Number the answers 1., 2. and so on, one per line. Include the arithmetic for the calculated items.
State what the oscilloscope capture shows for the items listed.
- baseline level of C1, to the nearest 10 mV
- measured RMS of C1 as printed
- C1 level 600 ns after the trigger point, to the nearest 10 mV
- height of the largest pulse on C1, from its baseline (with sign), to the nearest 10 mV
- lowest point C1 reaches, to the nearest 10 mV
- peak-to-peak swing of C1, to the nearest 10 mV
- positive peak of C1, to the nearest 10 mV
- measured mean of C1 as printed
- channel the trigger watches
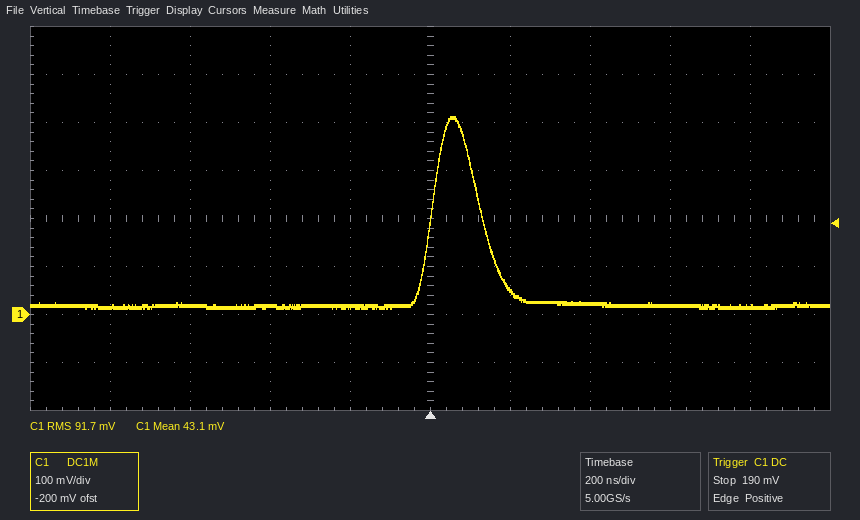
1. 20 mV
2. 91.7 mV
3. 20 mV
4. 410 mV − (20 mV) = +390 mV
5. 10 mV
6. 410 mV − (10 mV) = 400 mV
7. 410 mV
8. 43.1 mV
9. C1
